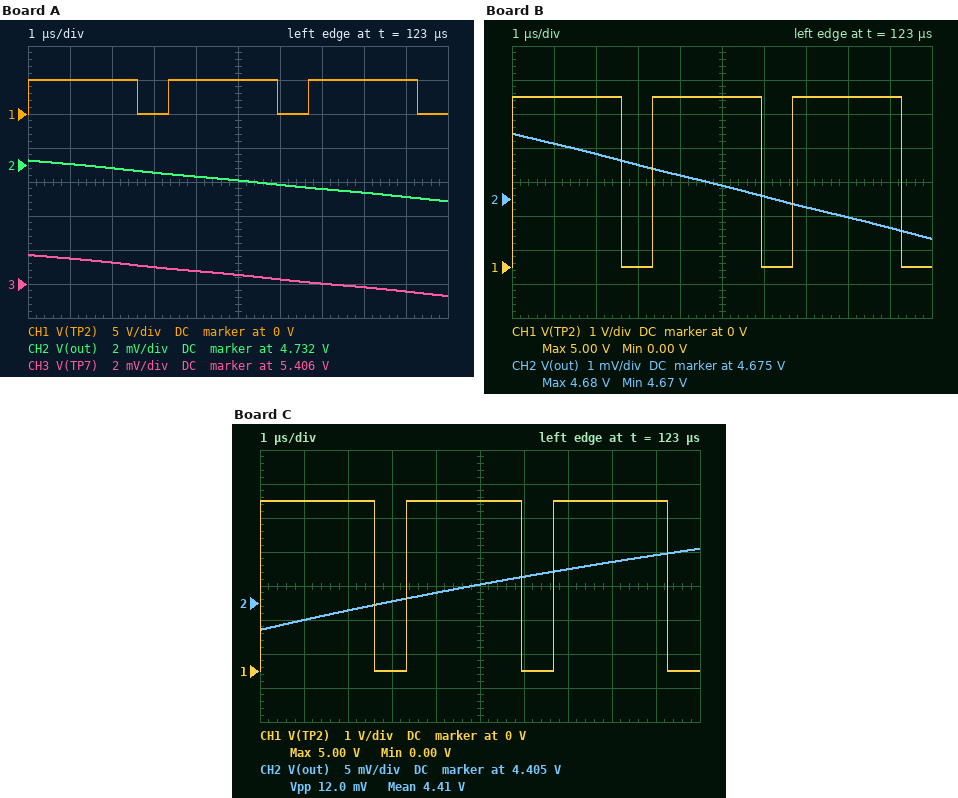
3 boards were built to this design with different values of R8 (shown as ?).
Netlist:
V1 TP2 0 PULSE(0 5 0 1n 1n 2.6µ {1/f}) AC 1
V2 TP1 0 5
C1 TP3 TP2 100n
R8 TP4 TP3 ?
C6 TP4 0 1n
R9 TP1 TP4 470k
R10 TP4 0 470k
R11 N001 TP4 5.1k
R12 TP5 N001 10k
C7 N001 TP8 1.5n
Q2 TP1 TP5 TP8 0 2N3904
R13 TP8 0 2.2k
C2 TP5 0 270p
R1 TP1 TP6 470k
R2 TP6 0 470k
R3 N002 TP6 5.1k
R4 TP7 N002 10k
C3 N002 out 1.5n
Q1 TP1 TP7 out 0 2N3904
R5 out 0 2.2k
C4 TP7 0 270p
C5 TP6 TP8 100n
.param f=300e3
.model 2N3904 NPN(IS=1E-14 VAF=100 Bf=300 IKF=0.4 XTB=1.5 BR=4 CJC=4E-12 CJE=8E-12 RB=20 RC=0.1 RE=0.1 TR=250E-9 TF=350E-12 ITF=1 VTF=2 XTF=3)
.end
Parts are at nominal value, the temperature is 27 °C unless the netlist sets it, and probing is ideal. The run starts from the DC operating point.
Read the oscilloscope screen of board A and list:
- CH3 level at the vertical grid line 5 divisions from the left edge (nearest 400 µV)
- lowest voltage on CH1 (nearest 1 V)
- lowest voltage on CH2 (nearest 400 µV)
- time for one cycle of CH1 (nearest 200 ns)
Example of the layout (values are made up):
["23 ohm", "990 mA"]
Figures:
["5.4064 V", "0 V", "4.7300 V", "3.4 µs"]
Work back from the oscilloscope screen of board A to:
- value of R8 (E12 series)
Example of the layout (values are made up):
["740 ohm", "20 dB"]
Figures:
["3.9 kΩ"]
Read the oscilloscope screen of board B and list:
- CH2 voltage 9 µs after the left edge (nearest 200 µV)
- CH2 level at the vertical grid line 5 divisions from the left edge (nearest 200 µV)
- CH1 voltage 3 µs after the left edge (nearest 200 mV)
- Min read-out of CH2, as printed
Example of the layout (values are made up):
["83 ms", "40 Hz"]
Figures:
["4.6742 V", "4.6754 V", "0 V", "4.67 V"]
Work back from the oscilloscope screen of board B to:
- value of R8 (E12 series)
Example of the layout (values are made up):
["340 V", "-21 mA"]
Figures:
["12 kΩ"]
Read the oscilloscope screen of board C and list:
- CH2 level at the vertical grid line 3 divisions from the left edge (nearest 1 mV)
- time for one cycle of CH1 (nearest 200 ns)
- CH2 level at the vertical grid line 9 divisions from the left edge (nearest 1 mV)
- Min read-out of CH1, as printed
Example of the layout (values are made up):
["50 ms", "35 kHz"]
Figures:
["4.405 V", "3.4 µs", "4.412 V", "0.00 V"]
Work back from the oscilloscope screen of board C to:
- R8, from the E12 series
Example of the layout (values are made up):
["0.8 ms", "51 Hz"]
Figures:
["27 kΩ"]
